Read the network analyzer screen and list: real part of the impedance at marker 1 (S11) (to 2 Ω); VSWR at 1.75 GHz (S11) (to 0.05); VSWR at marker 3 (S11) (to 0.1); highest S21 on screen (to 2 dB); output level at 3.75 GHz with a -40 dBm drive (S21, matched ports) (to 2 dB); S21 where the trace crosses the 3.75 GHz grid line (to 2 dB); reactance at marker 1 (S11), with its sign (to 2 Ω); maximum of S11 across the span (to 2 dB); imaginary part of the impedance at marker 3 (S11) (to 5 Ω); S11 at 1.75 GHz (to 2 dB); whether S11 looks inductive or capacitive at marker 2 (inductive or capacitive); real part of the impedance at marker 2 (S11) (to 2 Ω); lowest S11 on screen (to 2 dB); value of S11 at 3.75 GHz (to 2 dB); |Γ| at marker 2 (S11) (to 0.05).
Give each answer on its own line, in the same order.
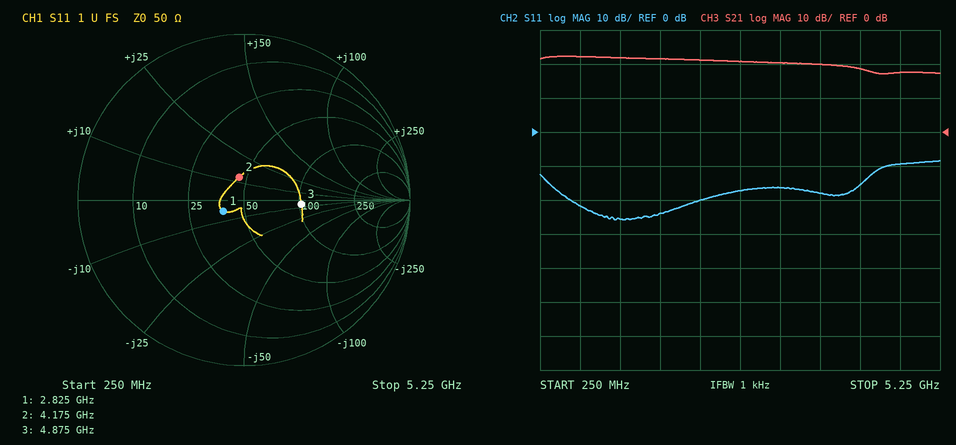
38 Ω
1.15
2.1
22 dB
-20 dBm
20 dB
-6 Ω
-8 dB
-5 Ω
-24 dB
inductive
46 Ω
-26 dB
-18 dB
0.15
